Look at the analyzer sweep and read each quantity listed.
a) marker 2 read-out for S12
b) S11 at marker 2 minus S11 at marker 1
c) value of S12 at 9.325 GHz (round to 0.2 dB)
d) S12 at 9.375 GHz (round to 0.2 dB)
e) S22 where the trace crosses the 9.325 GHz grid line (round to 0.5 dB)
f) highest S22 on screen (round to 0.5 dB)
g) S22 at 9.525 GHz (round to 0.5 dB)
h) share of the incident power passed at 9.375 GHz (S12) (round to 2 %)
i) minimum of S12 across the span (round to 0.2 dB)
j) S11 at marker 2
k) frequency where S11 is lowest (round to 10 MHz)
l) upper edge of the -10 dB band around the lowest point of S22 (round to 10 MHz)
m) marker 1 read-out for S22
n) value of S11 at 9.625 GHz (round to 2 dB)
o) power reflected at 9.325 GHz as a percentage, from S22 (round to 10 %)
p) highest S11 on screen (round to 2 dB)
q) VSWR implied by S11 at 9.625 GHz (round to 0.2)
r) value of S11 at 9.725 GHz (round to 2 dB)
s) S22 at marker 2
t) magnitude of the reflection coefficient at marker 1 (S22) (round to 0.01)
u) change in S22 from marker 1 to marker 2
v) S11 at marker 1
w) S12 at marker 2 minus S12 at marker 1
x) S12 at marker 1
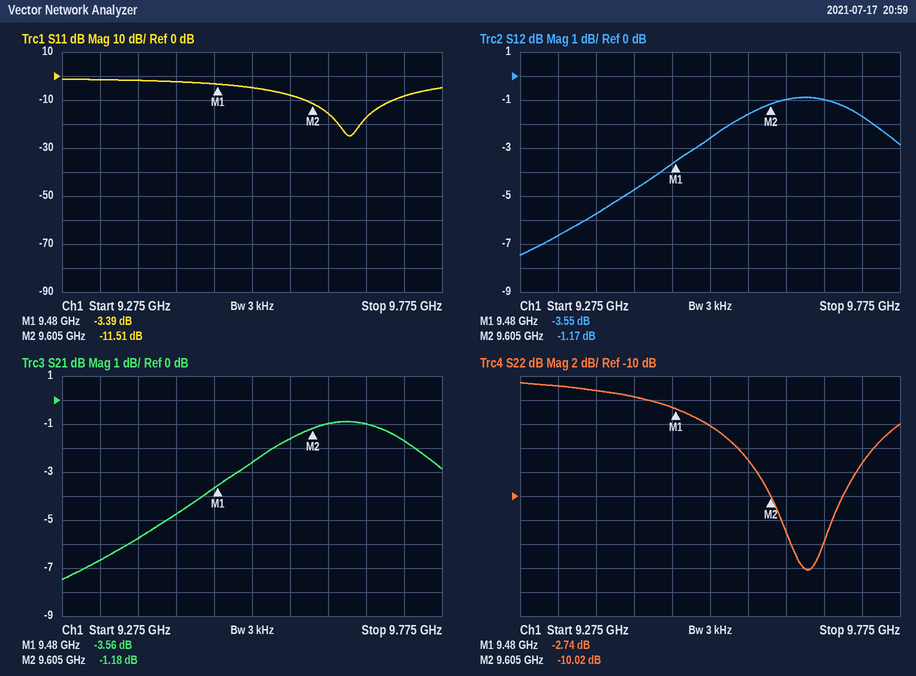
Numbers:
-1.17 dB
-8.12 dB
-6.6 dB
-5.8 dB
-1.0 dB
-0.5 dB
-4.0 dB
26 %
-7.4 dB
-11.51 dB
9.65 GHz
9.70 GHz
-2.74 dB
-16 dB
80 %
-2 dB
1.4
-8 dB
-10.02 dB
0.73
-7.28 dB
-3.39 dB
2.38 dB
-3.55 dB
